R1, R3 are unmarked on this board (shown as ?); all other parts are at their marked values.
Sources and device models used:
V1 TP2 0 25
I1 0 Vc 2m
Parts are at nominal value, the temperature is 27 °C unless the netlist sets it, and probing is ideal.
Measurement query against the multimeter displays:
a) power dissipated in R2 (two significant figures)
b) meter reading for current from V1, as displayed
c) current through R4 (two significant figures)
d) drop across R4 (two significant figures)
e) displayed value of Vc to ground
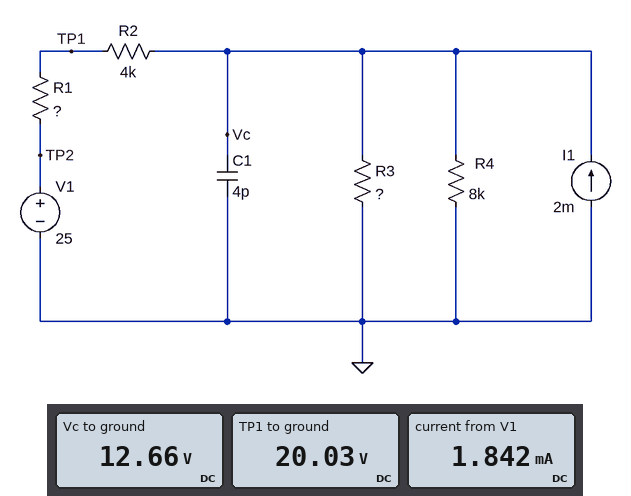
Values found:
14 mW
1.842 mA
1.6 mA
13 V
12.66 V
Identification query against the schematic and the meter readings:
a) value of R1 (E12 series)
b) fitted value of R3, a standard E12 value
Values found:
2.7 kΩ
5.6 kΩ
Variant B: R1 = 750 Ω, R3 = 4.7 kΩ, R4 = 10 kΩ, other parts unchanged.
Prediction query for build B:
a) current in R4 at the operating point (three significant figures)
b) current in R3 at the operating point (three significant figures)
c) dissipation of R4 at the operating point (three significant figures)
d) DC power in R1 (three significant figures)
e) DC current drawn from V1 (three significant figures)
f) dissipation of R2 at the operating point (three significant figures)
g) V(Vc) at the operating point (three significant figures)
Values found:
1.39 mA
2.95 mA
19.3 mW
4.11 mW
2.34 mA
21.9 mW
13.9 V
